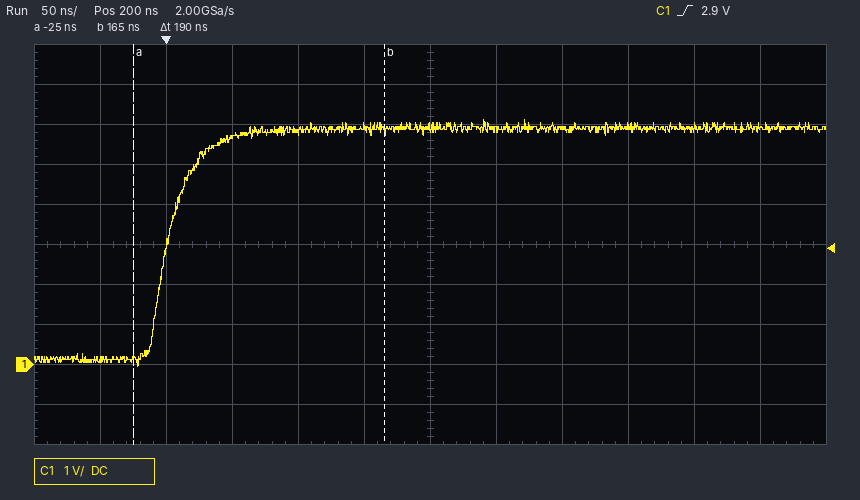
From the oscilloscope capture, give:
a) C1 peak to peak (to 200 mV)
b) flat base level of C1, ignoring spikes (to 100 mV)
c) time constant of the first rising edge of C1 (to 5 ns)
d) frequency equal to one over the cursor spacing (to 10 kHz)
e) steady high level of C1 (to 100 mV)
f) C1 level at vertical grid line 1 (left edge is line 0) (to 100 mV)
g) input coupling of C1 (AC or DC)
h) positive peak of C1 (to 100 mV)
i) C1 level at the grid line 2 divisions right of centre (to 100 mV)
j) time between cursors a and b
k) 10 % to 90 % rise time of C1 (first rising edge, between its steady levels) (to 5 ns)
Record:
6.2 V
100 mV
20 ns
5.26 MHz
5.9 V
100 mV
DC
6.1 V
5.9 V
190 ns
40 ns
